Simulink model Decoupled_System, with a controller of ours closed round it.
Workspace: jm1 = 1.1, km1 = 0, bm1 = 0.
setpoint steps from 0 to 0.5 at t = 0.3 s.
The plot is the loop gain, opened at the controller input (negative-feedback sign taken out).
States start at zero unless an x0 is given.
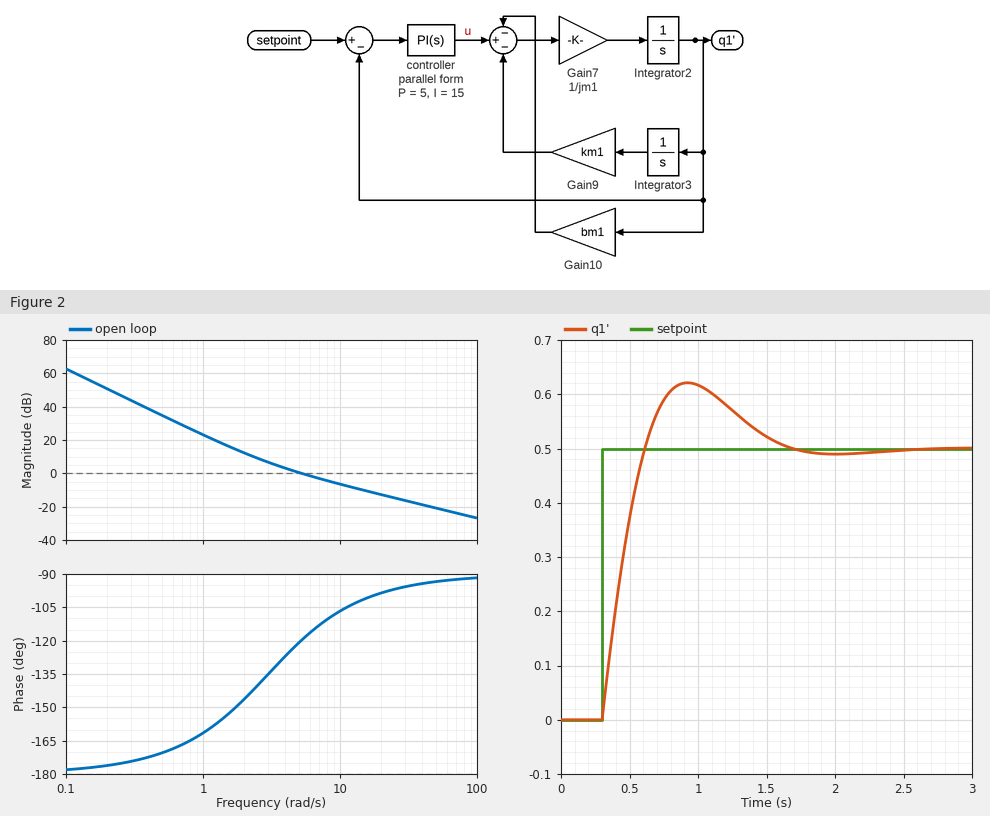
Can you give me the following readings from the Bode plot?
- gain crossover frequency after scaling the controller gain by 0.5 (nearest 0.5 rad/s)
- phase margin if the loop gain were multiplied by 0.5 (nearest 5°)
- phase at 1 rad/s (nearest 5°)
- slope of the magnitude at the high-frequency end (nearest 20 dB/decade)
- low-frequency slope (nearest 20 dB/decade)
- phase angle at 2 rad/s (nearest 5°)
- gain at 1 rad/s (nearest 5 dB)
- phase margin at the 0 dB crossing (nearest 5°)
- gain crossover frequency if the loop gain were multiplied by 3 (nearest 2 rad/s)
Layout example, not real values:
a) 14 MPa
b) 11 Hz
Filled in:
a) 3.0 rad/s
b) 45°
c) -160°
d) -20 dB/decade
e) -40 dB/decade
f) -145°
g) 25 dB
h) 60°
i) 14 rad/s
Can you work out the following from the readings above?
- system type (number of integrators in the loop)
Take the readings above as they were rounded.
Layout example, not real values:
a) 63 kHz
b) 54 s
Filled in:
a) 2
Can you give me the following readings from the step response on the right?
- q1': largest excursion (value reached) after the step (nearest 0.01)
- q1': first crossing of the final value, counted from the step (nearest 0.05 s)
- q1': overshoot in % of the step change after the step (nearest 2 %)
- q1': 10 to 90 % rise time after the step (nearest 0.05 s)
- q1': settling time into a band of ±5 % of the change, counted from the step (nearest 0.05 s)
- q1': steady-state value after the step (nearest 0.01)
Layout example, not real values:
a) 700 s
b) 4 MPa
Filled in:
a) 0.62
b) 0.30 s
c) 24 %
d) 0.25 s
e) 1.20 s
f) 0.50
